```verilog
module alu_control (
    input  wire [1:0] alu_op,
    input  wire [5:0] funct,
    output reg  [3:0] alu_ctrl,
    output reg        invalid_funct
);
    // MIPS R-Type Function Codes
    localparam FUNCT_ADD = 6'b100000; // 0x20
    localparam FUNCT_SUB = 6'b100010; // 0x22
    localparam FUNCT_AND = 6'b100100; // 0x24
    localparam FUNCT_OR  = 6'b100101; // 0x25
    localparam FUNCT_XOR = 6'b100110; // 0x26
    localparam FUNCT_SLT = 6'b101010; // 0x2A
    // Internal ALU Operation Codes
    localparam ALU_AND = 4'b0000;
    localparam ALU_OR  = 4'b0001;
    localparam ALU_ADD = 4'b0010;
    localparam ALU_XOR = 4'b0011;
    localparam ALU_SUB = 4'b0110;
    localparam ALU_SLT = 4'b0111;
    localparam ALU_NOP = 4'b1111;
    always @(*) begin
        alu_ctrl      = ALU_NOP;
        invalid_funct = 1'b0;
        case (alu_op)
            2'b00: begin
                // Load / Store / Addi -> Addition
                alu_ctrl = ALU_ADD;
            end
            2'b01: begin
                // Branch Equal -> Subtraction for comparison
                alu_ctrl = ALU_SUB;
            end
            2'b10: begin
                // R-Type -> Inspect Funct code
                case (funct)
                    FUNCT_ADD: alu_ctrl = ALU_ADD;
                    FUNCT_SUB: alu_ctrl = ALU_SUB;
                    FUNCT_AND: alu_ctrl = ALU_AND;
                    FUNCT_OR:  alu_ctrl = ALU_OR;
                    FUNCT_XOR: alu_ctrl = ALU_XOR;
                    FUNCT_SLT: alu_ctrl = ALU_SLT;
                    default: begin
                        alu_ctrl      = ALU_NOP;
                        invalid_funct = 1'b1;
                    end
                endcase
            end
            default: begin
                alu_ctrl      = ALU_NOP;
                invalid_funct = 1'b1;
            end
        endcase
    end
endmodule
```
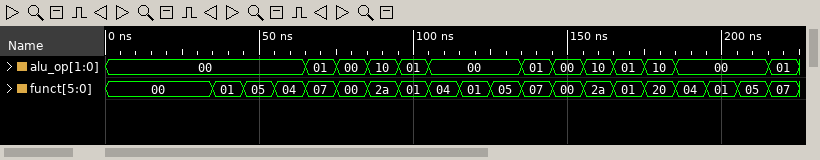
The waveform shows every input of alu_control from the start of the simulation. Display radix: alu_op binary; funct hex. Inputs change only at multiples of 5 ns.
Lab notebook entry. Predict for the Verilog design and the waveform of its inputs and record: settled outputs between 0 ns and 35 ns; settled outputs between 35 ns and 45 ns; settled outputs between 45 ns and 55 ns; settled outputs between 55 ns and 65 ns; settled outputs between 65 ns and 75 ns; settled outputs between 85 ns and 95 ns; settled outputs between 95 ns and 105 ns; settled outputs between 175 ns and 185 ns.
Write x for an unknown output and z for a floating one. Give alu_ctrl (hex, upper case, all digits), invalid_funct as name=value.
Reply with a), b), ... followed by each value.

a) alu_ctrl=2, invalid_funct=0
b) alu_ctrl=2, invalid_funct=0
c) alu_ctrl=2, invalid_funct=0
d) alu_ctrl=2, invalid_funct=0
e) alu_ctrl=6, invalid_funct=0
f) alu_ctrl=7, invalid_funct=0
g) alu_ctrl=6, invalid_funct=0
h) alu_ctrl=2, invalid_funct=0
